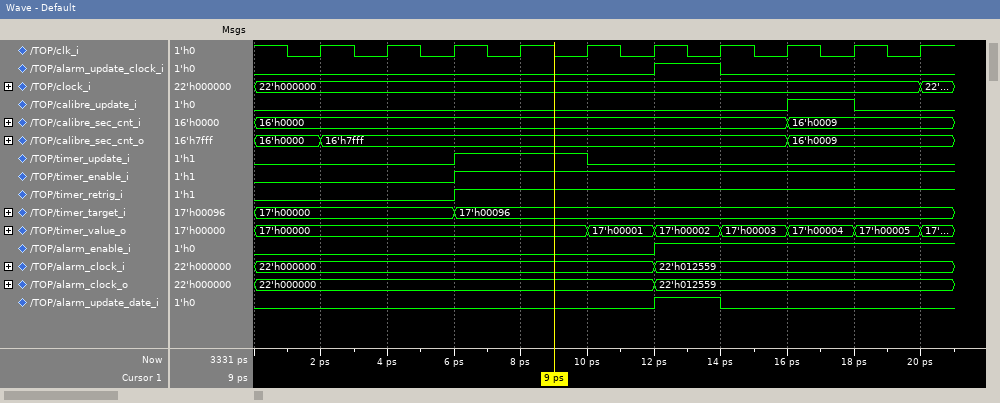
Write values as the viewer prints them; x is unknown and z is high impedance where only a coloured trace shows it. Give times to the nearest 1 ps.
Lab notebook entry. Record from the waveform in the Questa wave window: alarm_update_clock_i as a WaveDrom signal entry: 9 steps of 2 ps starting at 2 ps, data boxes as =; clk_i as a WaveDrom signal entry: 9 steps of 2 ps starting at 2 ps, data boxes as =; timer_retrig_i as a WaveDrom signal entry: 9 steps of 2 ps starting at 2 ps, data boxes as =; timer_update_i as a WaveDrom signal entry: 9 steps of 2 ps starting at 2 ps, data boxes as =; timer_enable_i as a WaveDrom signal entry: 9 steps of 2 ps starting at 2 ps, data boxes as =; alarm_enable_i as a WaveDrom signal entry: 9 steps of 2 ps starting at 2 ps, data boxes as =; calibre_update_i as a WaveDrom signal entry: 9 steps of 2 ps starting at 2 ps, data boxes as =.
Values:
{name: 'alarm_update_clock_i', wave: '0....10..'}
{name: 'clk_i', wave: 'p........'}
{name: 'timer_retrig_i', wave: '0.1......'}
{name: 'timer_update_i', wave: '0.1.0....'}
{name: 'timer_enable_i', wave: '0.1......'}
{name: 'alarm_enable_i', wave: '0....1...'}
{name: 'calibre_update_i', wave: '0......10'}
